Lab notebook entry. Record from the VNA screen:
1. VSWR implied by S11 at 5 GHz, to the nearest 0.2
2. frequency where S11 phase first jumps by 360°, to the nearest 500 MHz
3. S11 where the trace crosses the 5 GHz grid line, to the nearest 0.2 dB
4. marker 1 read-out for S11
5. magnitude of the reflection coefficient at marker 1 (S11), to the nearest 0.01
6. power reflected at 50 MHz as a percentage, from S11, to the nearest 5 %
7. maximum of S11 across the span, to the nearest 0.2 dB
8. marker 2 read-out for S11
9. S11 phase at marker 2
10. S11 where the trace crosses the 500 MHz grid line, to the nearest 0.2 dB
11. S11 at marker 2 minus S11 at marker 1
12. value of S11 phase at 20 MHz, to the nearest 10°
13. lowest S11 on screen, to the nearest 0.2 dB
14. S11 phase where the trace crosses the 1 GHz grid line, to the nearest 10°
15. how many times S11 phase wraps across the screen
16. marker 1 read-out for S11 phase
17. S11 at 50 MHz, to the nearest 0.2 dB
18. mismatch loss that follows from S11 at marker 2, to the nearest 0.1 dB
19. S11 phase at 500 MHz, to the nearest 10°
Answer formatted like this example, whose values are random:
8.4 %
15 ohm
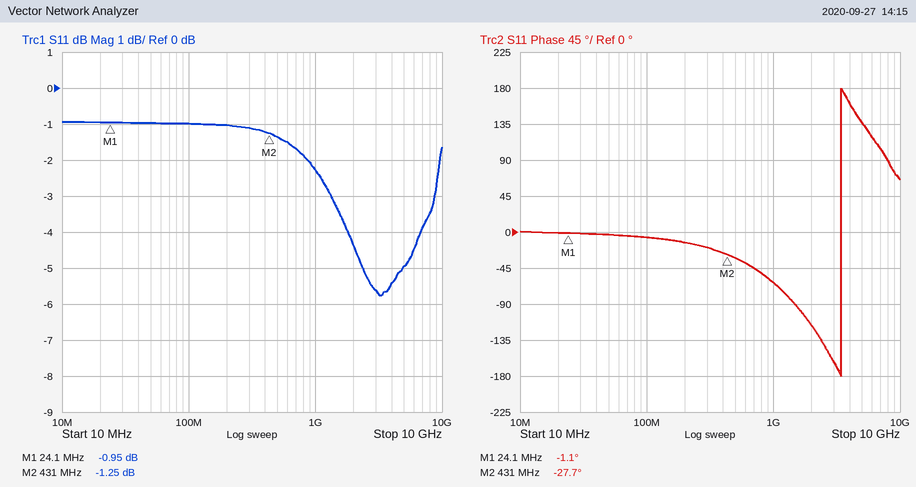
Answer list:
3.6
3.5 GHz
-5.0 dB
-0.95 dB
0.90
80 %
-1.0 dB
-1.25 dB
-27.7°
-1.4 dB
-0.30 dB
0°
-5.8 dB
-60°
1
-1.1°
-1.0 dB
6.0 dB
-30°
